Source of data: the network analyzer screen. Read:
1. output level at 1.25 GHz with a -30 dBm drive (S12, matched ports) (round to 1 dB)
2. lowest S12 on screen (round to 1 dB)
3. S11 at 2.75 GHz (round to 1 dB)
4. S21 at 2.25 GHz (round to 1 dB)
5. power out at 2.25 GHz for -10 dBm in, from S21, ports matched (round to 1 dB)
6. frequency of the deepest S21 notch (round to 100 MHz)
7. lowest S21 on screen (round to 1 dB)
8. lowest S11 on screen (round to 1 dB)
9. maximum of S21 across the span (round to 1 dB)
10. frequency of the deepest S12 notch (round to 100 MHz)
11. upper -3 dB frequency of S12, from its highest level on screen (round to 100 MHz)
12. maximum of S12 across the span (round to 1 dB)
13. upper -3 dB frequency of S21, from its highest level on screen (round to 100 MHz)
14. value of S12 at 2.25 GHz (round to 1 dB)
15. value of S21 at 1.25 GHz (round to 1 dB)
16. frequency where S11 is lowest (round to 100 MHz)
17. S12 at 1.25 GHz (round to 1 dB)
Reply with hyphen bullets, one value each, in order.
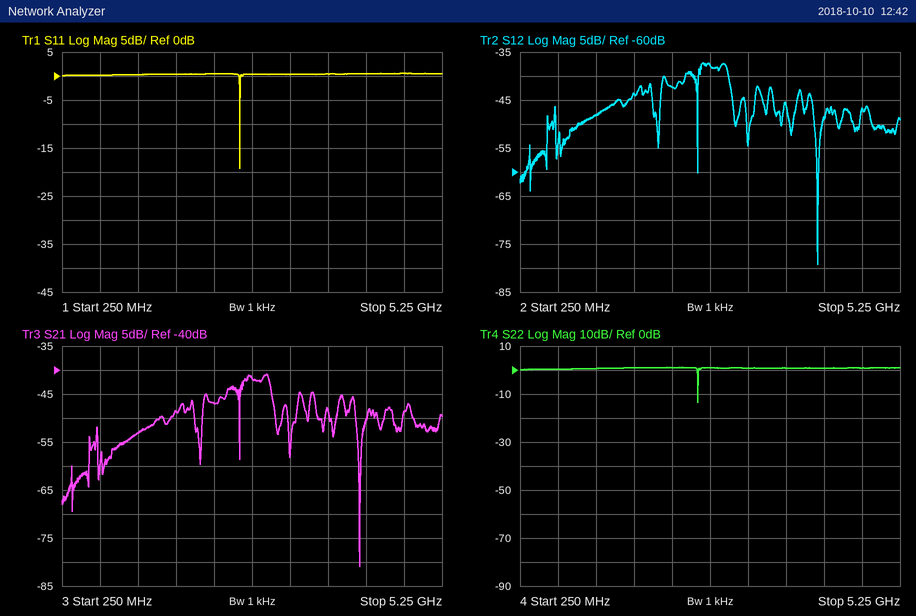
- -78 dBm
- -79 dB
- 0 dB
- -47 dB
- -57 dBm
- 4.2 GHz
- -81 dB
- -19 dB
- -41 dB
- 4.2 GHz
- 3.0 GHz
- -37 dB
- 3.0 GHz
- -42 dB
- -53 dB
- 2.6 GHz
- -48 dB
